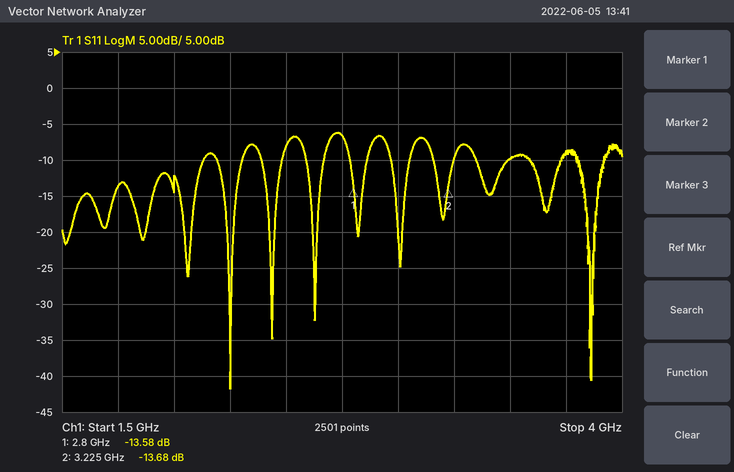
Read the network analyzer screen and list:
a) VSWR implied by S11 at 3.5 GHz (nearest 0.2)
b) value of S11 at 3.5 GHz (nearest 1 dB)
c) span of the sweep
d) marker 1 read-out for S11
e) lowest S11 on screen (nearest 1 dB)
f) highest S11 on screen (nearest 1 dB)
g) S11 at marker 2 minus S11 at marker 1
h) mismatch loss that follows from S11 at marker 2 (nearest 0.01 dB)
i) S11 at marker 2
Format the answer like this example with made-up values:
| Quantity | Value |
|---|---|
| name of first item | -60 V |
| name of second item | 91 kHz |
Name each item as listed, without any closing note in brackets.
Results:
| Quantity | Value |
|---|---|
| VSWR implied by S11 at 3.5 GHz | 2.0 |
| value of S11 at 3.5 GHz | -10 dB |
| span of the sweep | 2.5 GHz |
| marker 1 read-out for S11 | -13.58 dB |
| lowest S11 on screen | -42 dB |
| highest S11 on screen | -6 dB |
| S11 at marker 2 minus S11 at marker 1 | -0.10 dB |
| mismatch loss that follows from S11 at marker 2 | 0.19 dB |
| S11 at marker 2 | -13.68 dB |
